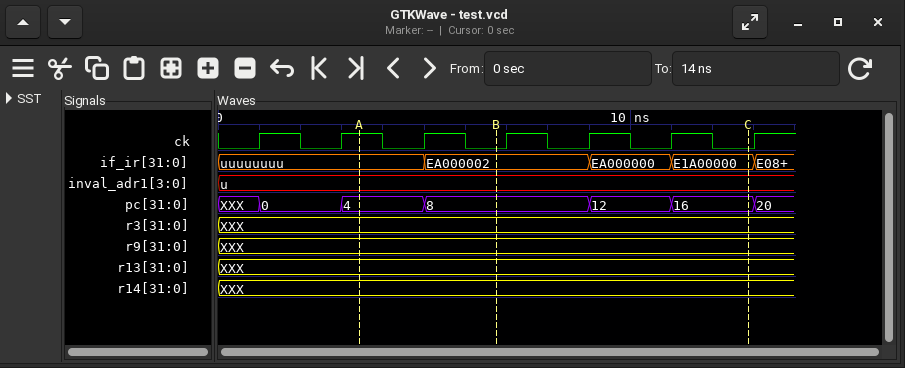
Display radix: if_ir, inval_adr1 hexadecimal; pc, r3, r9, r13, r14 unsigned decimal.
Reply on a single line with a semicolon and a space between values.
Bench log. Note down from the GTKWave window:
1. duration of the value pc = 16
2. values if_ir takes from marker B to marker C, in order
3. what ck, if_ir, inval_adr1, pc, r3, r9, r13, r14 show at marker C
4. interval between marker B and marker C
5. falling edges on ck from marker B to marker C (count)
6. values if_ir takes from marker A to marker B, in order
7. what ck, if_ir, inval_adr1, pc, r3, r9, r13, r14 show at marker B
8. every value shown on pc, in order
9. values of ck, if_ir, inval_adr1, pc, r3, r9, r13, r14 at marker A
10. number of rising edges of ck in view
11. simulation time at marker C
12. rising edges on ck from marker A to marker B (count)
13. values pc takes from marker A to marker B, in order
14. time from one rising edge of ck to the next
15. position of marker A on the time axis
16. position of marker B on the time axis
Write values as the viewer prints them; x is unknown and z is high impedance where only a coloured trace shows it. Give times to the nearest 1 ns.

2 ns; EA000002, EA000000, E1A00000; ck=0, if_ir=E1A00000, inval_adr1=u, pc=16, r3=XXX, r9=XXX, r13=XXX, r14=XXX; 6 ns; 3; uuuuuuuu, EA000002; ck=0, if_ir=EA000002, inval_adr1=u, pc=8, r3=XXX, r9=XXX, r13=XXX, r14=XXX; XXX, 0, 4, 8, 12, 16, 20; ck=1, if_ir=uuuuuuuu, inval_adr1=u, pc=4, r3=XXX, r9=XXX, r13=XXX, r14=XXX; 7; 13 ns; 1; 4, 8; 2 ns; 3 ns; 7 ns
